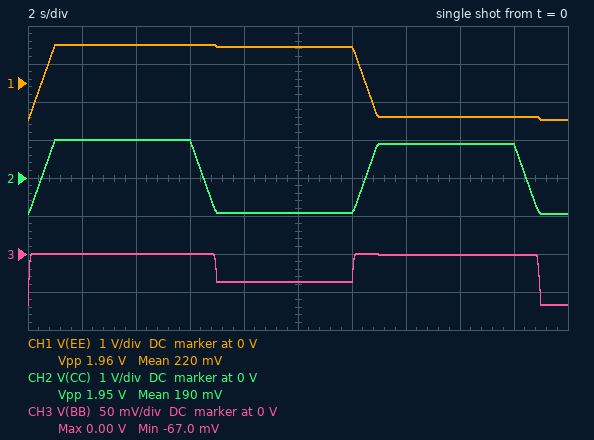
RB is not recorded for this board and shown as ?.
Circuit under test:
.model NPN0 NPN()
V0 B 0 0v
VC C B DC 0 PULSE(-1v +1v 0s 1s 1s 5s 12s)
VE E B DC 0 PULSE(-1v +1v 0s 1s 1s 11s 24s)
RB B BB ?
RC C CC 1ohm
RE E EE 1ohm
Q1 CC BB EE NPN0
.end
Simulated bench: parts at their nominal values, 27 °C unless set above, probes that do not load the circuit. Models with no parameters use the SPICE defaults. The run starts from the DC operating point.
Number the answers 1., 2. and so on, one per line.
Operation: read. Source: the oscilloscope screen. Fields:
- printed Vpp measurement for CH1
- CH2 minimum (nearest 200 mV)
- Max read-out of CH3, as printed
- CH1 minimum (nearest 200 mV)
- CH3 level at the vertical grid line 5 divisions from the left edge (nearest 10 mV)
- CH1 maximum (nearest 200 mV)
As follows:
1. 1.96 V
2. -1.0 V
3. 0.00 V
4. -1.0 V
5. -40 mV
6. 1.0 V
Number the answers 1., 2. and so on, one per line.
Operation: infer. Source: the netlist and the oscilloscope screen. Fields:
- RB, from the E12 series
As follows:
1. 0.82 Ω
